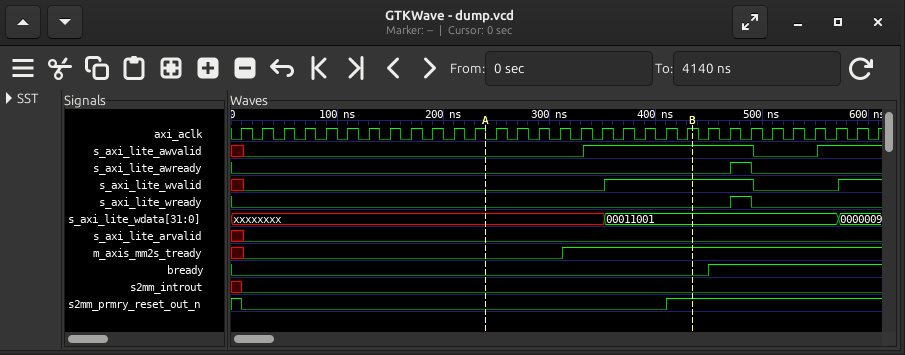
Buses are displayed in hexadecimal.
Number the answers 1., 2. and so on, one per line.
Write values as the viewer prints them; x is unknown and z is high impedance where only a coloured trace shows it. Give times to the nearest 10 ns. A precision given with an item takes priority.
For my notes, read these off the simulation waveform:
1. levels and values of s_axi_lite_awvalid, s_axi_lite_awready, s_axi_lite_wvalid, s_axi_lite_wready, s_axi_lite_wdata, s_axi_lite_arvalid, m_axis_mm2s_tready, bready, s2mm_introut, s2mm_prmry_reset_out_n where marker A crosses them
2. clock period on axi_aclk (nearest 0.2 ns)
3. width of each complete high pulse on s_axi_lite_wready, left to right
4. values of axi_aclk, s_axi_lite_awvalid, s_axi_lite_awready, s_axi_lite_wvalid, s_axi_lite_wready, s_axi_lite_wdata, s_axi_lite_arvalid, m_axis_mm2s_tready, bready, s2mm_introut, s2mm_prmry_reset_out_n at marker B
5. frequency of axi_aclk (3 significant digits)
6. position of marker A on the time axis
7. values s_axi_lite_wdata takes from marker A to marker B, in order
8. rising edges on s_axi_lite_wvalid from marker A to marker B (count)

1. s_axi_lite_awvalid=0, s_axi_lite_awready=0, s_axi_lite_wvalid=0, s_axi_lite_wready=0, s_axi_lite_wdata=xxxxxxxx, s_axi_lite_arvalid=0, m_axis_mm2s_tready=0, bready=0, s2mm_introut=0, s2mm_prmry_reset_out_n=0
2. 20 ns
3. 20 ns
4. axi_aclk=1, s_axi_lite_awvalid=1, s_axi_lite_awready=0, s_axi_lite_wvalid=1, s_axi_lite_wready=0, s_axi_lite_wdata=00011001, s_axi_lite_arvalid=0, m_axis_mm2s_tready=1, bready=0, s2mm_introut=0, s2mm_prmry_reset_out_n=1
5. 50.0 MHz
6. 240 ns
7. xxxxxxxx, 00011001
8. 1
